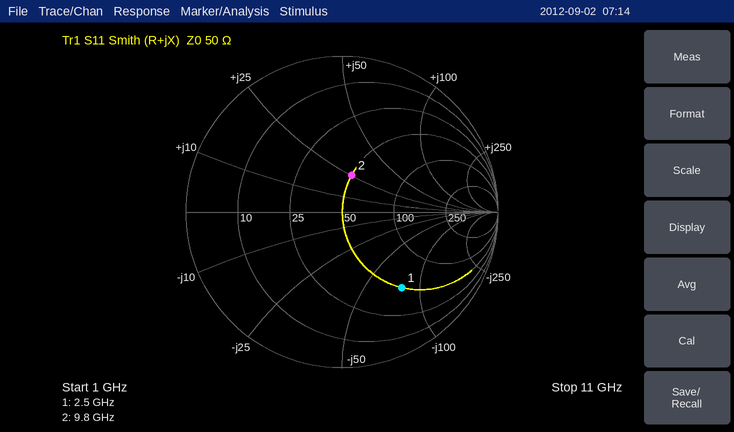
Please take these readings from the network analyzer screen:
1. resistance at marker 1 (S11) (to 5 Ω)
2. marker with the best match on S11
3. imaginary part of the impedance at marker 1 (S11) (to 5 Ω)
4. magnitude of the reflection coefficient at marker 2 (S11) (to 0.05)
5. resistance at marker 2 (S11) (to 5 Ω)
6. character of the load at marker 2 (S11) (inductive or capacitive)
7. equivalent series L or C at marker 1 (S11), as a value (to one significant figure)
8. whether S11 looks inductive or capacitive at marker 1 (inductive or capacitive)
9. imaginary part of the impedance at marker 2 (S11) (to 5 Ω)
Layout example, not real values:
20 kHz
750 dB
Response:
50 Ω
marker 2
-80 Ω
0.25
50 Ω
inductive
800 fF
capacitive
+25 Ω
